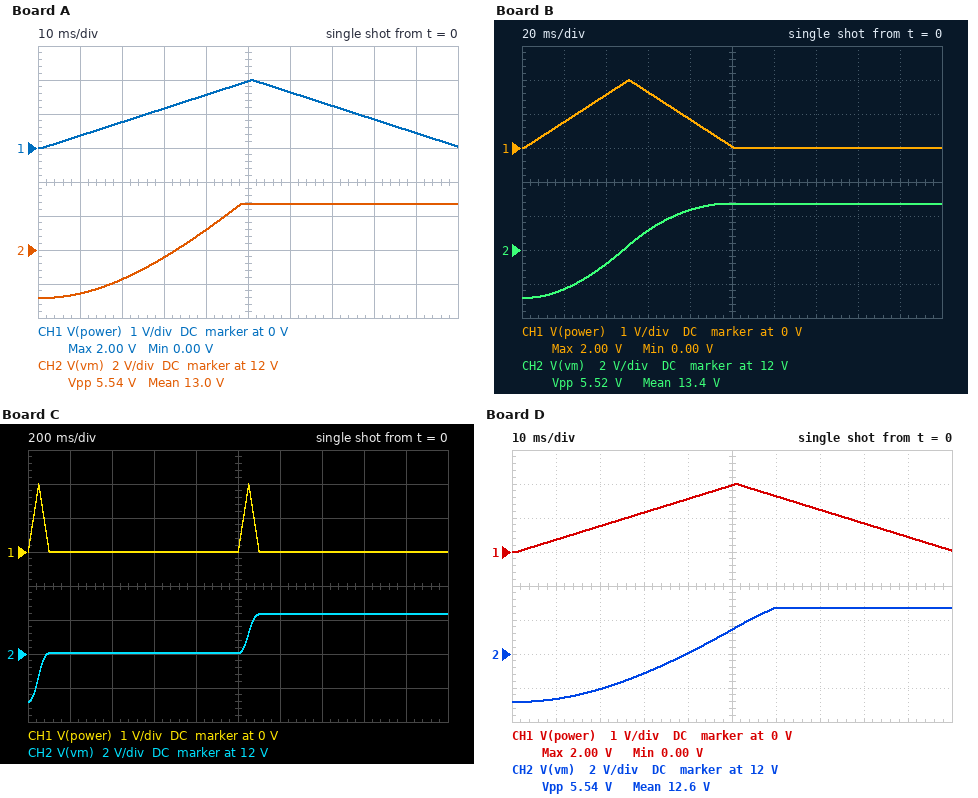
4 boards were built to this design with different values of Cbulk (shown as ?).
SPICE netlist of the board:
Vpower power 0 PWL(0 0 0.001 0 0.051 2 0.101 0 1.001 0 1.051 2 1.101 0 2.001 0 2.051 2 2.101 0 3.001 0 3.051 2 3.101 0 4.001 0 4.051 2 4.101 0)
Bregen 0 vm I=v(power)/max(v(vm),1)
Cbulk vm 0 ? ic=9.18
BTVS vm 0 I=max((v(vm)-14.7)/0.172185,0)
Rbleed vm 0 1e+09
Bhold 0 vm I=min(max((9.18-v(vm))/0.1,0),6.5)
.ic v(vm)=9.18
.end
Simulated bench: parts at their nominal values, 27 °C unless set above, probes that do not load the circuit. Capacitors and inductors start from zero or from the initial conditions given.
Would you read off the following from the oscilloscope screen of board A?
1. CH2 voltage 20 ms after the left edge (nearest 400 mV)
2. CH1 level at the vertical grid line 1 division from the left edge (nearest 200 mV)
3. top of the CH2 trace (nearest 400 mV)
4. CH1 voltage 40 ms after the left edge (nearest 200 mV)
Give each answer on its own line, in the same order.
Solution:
10.4 V
400 mV
14.8 V
1.6 V
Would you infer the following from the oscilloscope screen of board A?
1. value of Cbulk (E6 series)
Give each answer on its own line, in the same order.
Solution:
680 µF
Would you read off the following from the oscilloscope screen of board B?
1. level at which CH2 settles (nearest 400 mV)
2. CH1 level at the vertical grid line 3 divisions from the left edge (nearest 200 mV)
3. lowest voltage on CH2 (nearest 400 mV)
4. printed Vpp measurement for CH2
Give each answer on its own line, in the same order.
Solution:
14.8 V
1.6 V
9.2 V
5.52 V
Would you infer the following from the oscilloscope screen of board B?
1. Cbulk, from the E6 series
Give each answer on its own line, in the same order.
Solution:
1.5 mF
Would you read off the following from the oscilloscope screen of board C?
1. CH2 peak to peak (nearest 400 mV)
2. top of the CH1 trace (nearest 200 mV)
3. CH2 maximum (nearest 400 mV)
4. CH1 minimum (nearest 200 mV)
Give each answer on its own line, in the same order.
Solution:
5.2 V
2.0 V
14.4 V
0 V
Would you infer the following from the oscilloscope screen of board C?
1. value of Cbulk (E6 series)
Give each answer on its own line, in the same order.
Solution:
3.3 mF
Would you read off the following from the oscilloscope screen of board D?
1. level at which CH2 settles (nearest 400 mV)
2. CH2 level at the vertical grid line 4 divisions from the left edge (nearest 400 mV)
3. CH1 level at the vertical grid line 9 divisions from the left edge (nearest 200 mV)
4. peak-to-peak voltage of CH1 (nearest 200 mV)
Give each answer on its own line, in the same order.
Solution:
14.8 V
12.0 V
400 mV
2.0 V
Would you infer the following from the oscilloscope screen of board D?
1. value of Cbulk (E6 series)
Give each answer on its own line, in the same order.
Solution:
1 mF
